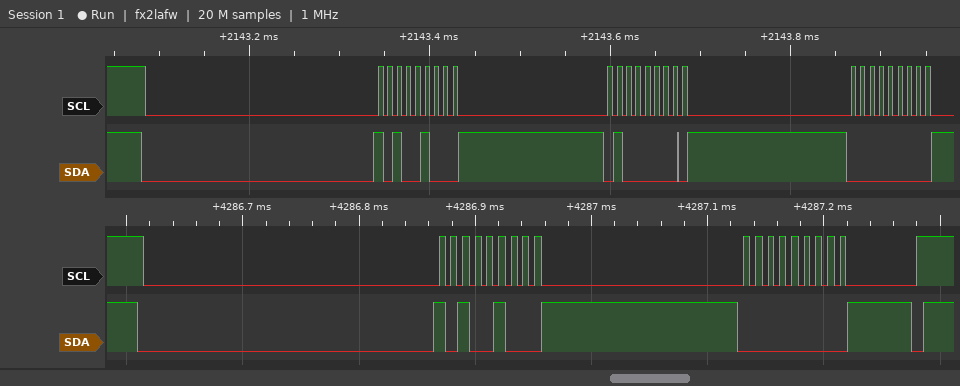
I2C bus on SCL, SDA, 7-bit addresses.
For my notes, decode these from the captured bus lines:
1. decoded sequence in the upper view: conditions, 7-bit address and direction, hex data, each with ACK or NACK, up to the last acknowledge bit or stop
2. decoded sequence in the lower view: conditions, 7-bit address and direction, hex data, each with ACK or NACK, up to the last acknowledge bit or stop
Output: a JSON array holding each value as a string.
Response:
["start, address 52 write ACK, 40 ACK, 00 ACK", "start, address 52 write ACK, 00 ACK, stop"]
